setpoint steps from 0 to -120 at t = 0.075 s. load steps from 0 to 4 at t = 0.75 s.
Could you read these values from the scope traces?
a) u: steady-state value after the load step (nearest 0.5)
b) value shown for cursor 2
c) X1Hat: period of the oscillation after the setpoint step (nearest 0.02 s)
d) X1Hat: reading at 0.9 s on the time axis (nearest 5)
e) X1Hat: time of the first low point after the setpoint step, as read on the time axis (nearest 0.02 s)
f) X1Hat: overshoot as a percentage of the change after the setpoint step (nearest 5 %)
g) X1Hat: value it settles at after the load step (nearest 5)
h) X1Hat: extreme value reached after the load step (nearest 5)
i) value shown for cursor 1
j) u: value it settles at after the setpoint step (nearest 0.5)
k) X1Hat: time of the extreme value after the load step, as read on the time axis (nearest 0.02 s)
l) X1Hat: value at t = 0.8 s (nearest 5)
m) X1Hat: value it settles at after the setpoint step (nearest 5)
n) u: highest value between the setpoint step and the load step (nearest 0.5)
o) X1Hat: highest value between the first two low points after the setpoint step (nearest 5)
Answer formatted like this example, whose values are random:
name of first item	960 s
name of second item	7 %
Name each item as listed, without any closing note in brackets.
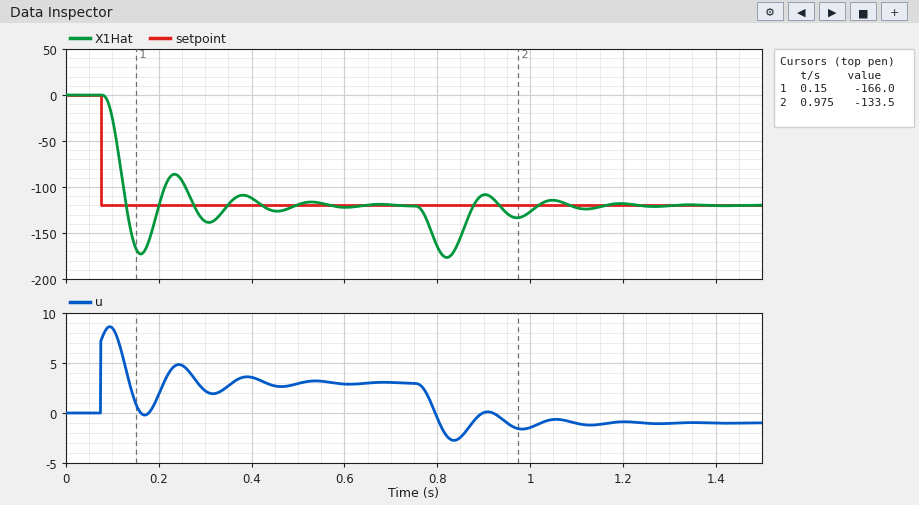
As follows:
u: steady-state value after the load step	-1.0
value shown for cursor 2	-133.5
X1Hat: period of the oscillation after the setpoint step	0.14 s
X1Hat: reading at 0.9 s on the time axis	-110
X1Hat: time of the first low point after the setpoint step, as read on the time axis	0.16 s
X1Hat: overshoot as a percentage of the change after the setpoint step	45 %
X1Hat: value it settles at after the load step	-120
X1Hat: extreme value reached after the load step	-175
value shown for cursor 1	-166.0
u: value it settles at after the setpoint step	3.0
X1Hat: time of the extreme value after the load step, as read on the time axis	0.82 s
X1Hat: value at t = 0.8 s	-165
X1Hat: value it settles at after the setpoint step	-120
u: highest value between the setpoint step and the load step	8.5
X1Hat: highest value between the first two low points after the setpoint step	-85
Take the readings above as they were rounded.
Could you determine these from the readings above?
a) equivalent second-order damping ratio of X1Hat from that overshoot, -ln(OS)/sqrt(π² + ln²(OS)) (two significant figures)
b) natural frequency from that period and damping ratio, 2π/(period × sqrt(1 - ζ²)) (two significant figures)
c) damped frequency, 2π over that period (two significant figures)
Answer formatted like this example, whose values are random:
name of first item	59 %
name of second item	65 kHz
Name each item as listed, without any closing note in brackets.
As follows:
equivalent second-order damping ratio of X1Hat from that overshoot, -ln(OS)/sqrt(π² + ln²(OS))	0.25
natural frequency from that period and damping ratio, 2π/(period × sqrt(1 - ζ²))	46 rad/s
damped frequency, 2π over that period	45 rad/s
